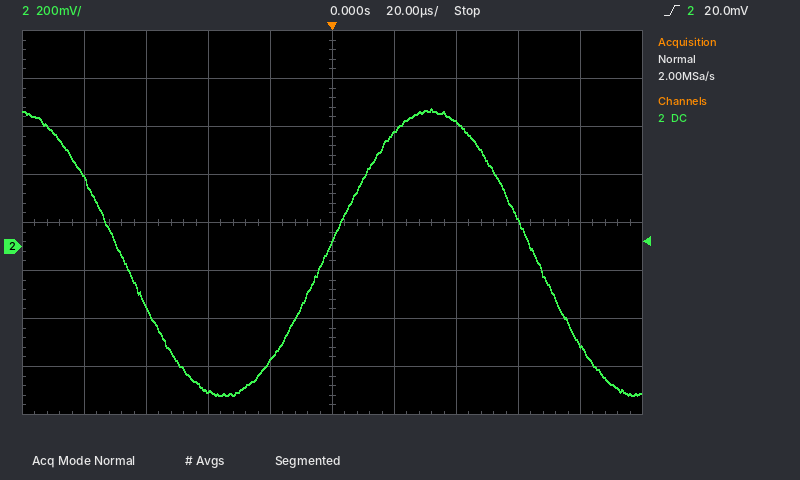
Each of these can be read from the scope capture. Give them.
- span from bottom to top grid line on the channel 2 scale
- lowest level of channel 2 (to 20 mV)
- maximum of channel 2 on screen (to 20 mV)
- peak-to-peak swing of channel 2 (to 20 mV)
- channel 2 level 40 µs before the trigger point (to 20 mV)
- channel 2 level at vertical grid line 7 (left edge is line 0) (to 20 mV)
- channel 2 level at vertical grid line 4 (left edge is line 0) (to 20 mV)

1.6 V
-620 mV
580 mV
1.20 V
-600 mV
520 mV
-480 mV
